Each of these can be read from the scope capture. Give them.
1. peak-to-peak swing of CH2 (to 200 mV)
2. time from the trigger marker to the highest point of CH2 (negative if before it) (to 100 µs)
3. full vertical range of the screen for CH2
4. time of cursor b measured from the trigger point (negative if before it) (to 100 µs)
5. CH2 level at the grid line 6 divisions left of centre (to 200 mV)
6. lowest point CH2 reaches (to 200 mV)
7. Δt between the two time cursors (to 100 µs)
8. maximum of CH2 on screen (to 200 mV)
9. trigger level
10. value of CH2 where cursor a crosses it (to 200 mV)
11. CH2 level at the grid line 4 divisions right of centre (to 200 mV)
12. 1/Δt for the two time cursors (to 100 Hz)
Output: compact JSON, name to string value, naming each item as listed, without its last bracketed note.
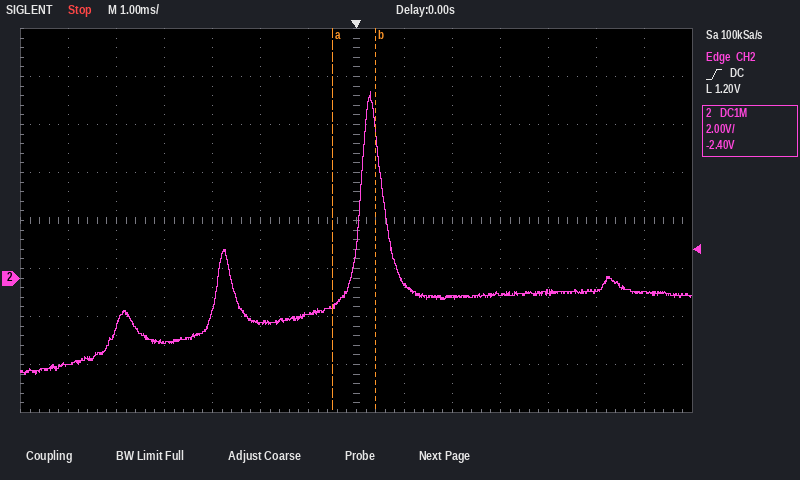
{"peak-to-peak swing of CH2": "11.8 V", "time from the trigger marker to the highest point of CH2 (negative if before it)": "+300 µs", "full vertical range of the screen for CH2": "16 V", "time of cursor b measured from the trigger point (negative if before it)": "+400 µs", "CH2 level at the grid line 6 divisions left of centre": "-3.6 V", "lowest point CH2 reaches": "-4.0 V", "Δt between the two time cursors": "900 µs", "maximum of CH2 on screen": "7.8 V", "trigger level": "1.20 V", "value of CH2 where cursor a crosses it": "-1.2 V", "CH2 level at the grid line 4 divisions right of centre": "-600 mV", "1/Δt for the two time cursors": "1.1 kHz"}
